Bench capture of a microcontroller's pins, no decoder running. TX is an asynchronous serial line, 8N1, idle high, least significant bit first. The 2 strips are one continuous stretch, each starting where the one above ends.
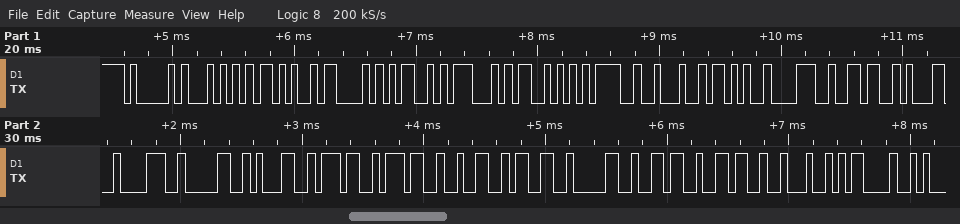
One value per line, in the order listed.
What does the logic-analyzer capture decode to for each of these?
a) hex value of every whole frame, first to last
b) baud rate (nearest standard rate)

41 54 2B 43 4D 47 53 3D 22 2B 38 36 31 38 30 31 37 37 32 33 30 36 36 22 0D
19200 baud
